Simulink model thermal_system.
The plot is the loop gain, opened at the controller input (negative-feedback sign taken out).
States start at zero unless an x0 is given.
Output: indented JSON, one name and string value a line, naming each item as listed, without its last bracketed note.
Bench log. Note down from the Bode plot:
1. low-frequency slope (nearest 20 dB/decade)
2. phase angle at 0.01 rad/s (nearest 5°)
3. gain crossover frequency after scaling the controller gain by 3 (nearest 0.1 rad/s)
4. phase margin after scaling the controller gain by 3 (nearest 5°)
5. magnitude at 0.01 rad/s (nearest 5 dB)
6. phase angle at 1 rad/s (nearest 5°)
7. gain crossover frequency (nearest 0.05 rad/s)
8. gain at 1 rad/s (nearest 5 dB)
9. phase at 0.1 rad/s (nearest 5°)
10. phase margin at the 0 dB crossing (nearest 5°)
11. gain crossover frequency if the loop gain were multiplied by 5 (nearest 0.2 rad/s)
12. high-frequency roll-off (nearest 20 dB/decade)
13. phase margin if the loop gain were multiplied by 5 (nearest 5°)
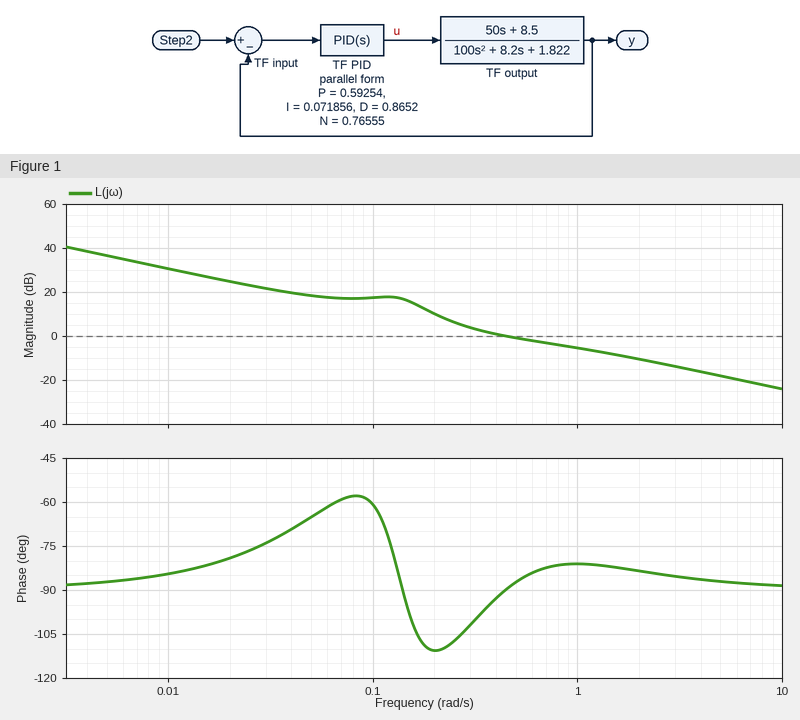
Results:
{
  "low-frequency slope": "-20 dB/decade",
  "phase angle at 0.01 rad/s": "-85°",
  "gain crossover frequency after scaling the controller gain by 3": "1.8 rad/s",
  "phase margin after scaling the controller gain by 3": "95°",
  "magnitude at 0.01 rad/s": "30 dB",
  "phase angle at 1 rad/s": "-80°",
  "gain crossover frequency": "0.45 rad/s",
  "gain at 1 rad/s": "-5 dB",
  "phase at 0.1 rad/s": "-60°",
  "phase margin at the 0 dB crossing": "90°",
  "gain crossover frequency if the loop gain were multiplied by 5": "3.0 rad/s",
  "high-frequency roll-off": "-20 dB/decade",
  "phase margin if the loop gain were multiplied by 5": "95°"
}
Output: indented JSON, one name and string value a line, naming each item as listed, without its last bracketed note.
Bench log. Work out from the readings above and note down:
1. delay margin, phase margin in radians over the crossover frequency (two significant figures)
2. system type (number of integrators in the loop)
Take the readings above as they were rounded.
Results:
{
  "delay margin, phase margin in radians over the crossover frequency": "3.5 s",
  "system type": "1"
}
